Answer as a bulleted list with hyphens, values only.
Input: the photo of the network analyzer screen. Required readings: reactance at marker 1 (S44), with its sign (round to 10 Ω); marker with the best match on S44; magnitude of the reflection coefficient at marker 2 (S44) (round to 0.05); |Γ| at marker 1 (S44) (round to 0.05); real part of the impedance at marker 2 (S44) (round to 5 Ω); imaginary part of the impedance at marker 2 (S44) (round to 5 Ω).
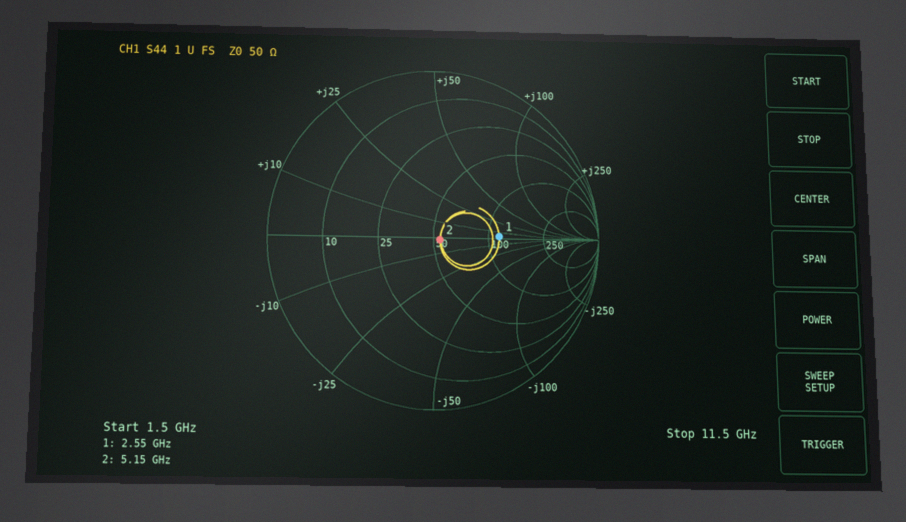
- 0 Ω
- marker 2
- 0.05
- 0.40
- 55 Ω
- 0 Ω
